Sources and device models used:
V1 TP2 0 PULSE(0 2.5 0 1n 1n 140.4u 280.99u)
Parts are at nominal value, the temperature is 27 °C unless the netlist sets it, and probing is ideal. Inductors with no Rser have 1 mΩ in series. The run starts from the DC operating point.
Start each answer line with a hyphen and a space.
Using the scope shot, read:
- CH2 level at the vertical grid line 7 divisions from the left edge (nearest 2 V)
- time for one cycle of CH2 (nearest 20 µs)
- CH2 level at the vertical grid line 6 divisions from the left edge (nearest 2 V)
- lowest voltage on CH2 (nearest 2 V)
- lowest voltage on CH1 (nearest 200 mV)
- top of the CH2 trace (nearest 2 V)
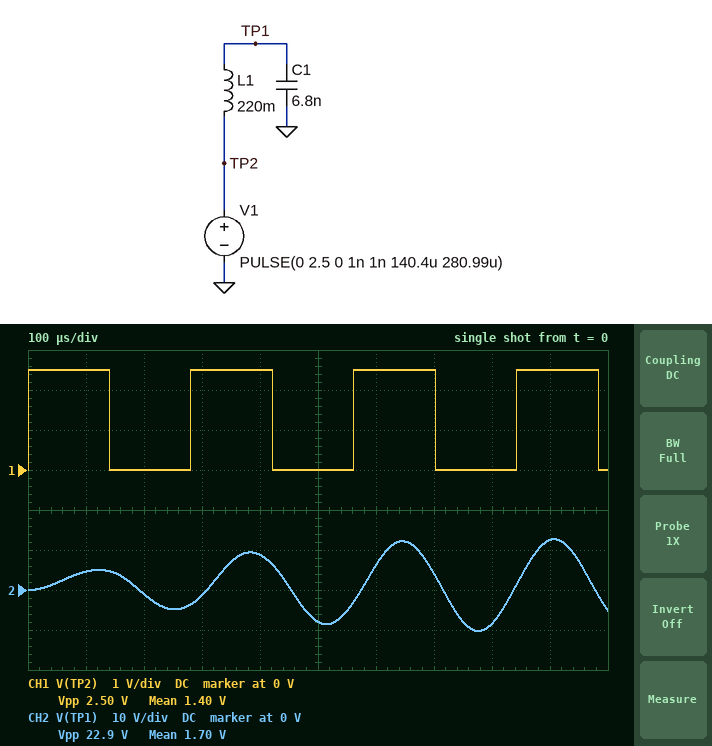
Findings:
- 4 V
- 260 µs
- 6 V
- -10 V
- 0 V
- 12 V
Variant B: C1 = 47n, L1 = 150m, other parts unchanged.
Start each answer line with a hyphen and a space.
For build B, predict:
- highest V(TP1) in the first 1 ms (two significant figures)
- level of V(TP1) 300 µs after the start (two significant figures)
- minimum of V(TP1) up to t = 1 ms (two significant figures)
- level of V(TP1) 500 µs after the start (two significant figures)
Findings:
- 3.7 V
- 1.5 V
- -900 mV
- 230 mV
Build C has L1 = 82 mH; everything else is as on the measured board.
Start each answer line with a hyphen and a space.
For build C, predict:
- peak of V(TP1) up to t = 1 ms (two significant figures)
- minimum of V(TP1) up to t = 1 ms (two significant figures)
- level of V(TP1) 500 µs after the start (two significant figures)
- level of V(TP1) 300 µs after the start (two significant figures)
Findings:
- 5.0 V
- -2.2 V
- -490 mV
- 510 mV
